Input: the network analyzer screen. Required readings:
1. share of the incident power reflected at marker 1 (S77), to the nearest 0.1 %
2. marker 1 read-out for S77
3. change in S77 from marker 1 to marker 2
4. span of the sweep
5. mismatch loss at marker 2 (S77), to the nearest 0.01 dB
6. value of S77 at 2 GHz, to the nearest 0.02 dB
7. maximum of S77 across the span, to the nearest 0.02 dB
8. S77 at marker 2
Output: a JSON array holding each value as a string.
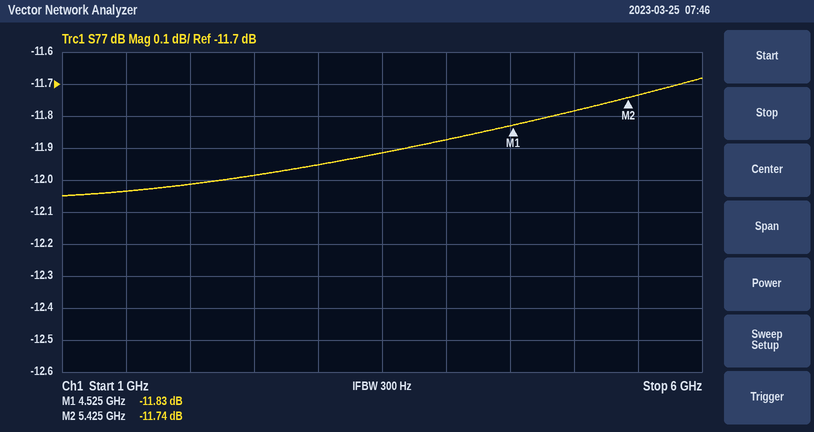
["6.6 %", "-11.83 dB", "0.09 dB", "5 GHz", "0.30 dB", "-12.02 dB", "-11.68 dB", "-11.74 dB"]
